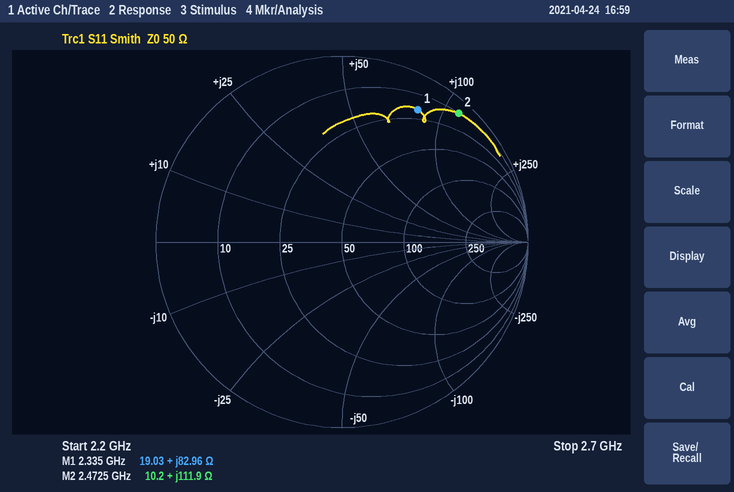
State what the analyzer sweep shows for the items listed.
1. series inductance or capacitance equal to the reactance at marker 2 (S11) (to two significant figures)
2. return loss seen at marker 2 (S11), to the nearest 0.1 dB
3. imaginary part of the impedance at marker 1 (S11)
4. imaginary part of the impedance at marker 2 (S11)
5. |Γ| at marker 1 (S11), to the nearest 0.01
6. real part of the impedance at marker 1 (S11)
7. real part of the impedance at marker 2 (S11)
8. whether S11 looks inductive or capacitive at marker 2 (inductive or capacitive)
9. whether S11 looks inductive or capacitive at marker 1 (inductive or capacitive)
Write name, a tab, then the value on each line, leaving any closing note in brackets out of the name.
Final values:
series inductance or capacitance equal to the reactance at marker 2 (S11)	7.2 nH
return loss seen at marker 2 (S11), to the nearest 0.1 dB	0.6 dB
imaginary part of the impedance at marker 1	+82.96 Ω
imaginary part of the impedance at marker 2	+111.9 Ω
|Γ| at marker 1 (S11), to the nearest 0.01	0.82
real part of the impedance at marker 1	19.03 Ω
real part of the impedance at marker 2	10.2 Ω
whether S11 looks inductive or capacitive at marker 2	inductive
whether S11 looks inductive or capacitive at marker 1	inductive
